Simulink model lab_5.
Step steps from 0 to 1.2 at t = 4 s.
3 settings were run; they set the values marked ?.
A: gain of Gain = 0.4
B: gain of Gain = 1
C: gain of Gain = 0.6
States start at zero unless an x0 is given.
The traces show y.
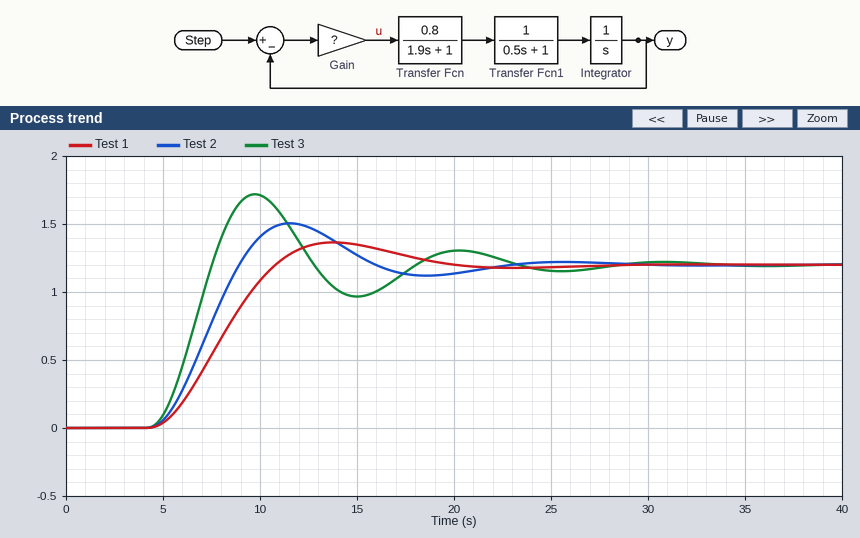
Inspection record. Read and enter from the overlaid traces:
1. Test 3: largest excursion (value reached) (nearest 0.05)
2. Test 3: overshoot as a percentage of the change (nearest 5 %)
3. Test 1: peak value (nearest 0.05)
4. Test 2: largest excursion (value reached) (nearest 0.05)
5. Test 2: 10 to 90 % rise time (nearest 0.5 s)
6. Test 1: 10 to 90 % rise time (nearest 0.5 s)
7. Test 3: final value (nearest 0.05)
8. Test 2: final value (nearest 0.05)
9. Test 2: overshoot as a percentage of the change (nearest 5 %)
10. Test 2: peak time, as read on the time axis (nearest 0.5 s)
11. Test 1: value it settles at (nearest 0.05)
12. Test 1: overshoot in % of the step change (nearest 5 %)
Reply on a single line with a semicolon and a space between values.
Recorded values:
1.70; 45 %; 1.35; 1.50; 3.0 s; 4.5 s; 1.20; 1.20; 25 %; 11.5 s; 1.20; 15 %
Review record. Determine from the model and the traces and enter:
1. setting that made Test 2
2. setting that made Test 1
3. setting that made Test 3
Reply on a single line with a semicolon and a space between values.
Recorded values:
C; A; B
